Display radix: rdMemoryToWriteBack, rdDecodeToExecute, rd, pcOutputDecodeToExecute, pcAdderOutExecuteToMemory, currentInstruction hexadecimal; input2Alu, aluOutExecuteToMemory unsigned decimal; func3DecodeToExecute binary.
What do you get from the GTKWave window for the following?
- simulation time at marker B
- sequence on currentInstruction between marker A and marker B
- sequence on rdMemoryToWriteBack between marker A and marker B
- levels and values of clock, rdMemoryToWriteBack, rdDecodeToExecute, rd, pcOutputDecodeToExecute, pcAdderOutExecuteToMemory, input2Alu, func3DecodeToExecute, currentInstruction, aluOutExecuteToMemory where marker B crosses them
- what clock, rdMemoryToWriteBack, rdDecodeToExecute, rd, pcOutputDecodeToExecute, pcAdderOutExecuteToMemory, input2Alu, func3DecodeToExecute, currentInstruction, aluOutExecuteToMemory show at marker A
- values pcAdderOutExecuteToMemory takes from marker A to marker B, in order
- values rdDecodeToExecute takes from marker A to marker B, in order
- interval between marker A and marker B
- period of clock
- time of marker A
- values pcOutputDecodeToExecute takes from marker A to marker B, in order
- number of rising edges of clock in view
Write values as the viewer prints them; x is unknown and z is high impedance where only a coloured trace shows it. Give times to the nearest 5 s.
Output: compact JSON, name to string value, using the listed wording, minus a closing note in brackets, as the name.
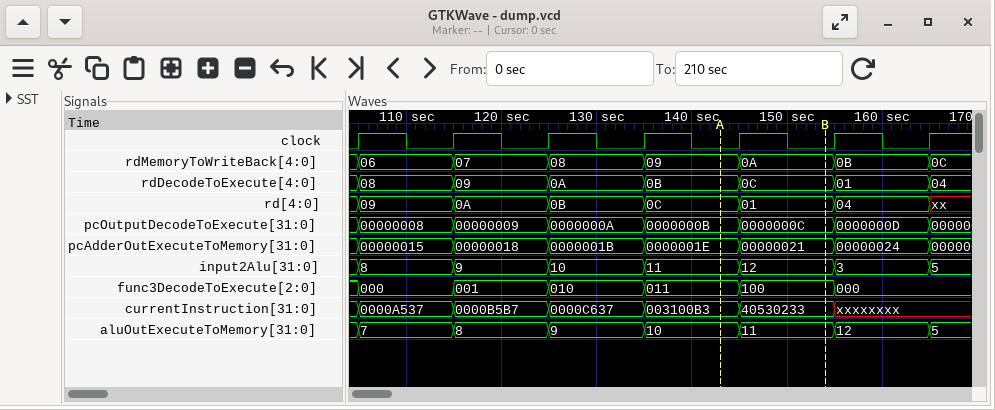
{"simulation time at marker B": "155 s", "sequence on currentInstruction between marker A and marker B": "003100B3, 40530233", "sequence on rdMemoryToWriteBack between marker A and marker B": "09, 0A", "levels and values of clock, rdMemoryToWriteBack, rdDecodeToExecute, rd, pcOutputDecodeToExecute, pcAdderOutExecuteToMemory, input2Alu, func3DecodeToExecute, currentInstruction, aluOutExecuteToMemory where marker B crosses them": "clock=0, rdMemoryToWriteBack=0A, rdDecodeToExecute=0C, rd=01, pcOutputDecodeToExecute=0000000C, pcAdderOutExecuteToMemory=00000021, input2Alu=12, func3DecodeToExecute=100, currentInstruction=40530233, aluOutExecuteToMemory=11", "what clock, rdMemoryToWriteBack, rdDecodeToExecute, rd, pcOutputDecodeToExecute, pcAdderOutExecuteToMemory, input2Alu, func3DecodeToExecute, currentInstruction, aluOutExecuteToMemory show at marker A": "clock=0, rdMemoryToWriteBack=09, rdDecodeToExecute=0B, rd=0C, pcOutputDecodeToExecute=0000000B, pcAdderOutExecuteToMemory=0000001E, input2Alu=11, func3DecodeToExecute=011, currentInstruction=003100B3, aluOutExecuteToMemory=10", "values pcAdderOutExecuteToMemory takes from marker A to marker B, in order": "0000001E, 00000021", "values rdDecodeToExecute takes from marker A to marker B, in order": "0B, 0C", "interval between marker A and marker B": "10 s", "period of clock": "10 s", "time of marker A": "145 s", "values pcOutputDecodeToExecute takes from marker A to marker B, in order": "0000000B, 0000000C", "number of rising edges of clock in view": "7"}
